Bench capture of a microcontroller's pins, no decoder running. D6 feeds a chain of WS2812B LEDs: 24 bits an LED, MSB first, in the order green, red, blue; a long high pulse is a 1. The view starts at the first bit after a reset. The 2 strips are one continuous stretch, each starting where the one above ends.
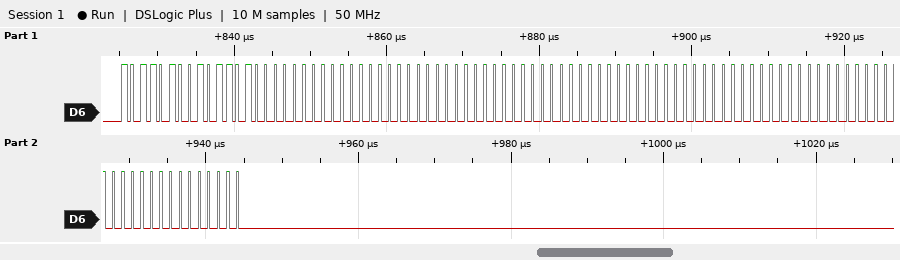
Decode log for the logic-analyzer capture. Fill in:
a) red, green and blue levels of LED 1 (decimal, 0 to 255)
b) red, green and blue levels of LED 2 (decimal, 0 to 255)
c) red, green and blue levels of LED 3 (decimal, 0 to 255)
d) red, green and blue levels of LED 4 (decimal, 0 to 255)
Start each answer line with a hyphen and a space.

- 180, 180, 0
- 0, 0, 0
- 0, 0, 0
- 0, 0, 0
